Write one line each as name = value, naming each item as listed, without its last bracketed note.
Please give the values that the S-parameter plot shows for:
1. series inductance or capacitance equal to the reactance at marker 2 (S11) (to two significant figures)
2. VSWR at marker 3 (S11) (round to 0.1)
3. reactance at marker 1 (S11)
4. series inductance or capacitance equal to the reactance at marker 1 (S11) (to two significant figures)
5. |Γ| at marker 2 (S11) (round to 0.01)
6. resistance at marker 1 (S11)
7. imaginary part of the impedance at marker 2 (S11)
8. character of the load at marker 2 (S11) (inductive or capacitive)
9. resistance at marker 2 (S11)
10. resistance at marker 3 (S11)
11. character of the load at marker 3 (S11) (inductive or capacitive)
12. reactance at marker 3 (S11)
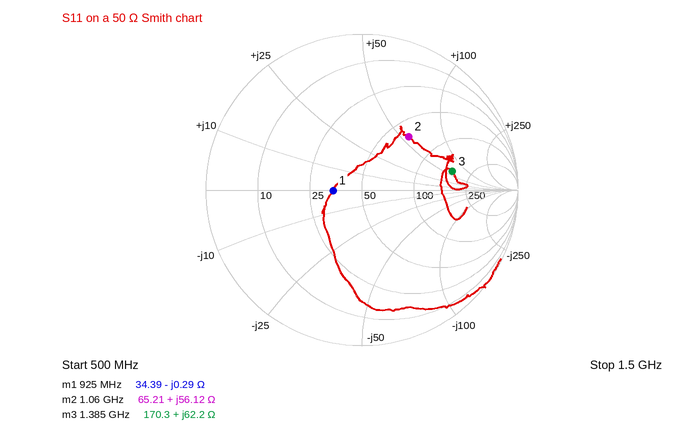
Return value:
series inductance or capacitance equal to the reactance at marker 2 (S11) = 8.4 nH
VSWR at marker 3 (S11) = 3.9
reactance at marker 1 = -0.29 Ω
series inductance or capacitance equal to the reactance at marker 1 (S11) = 590 pF
|Γ| at marker 2 (S11) = 0.45
resistance at marker 1 = 34.39 Ω
imaginary part of the impedance at marker 2 = +56.12 Ω
character of the load at marker 2 (S11) = inductive
resistance at marker 2 = 65.21 Ω
resistance at marker 3 = 170.3 Ω
character of the load at marker 3 (S11) = inductive
reactance at marker 3 = +62.2 Ω
